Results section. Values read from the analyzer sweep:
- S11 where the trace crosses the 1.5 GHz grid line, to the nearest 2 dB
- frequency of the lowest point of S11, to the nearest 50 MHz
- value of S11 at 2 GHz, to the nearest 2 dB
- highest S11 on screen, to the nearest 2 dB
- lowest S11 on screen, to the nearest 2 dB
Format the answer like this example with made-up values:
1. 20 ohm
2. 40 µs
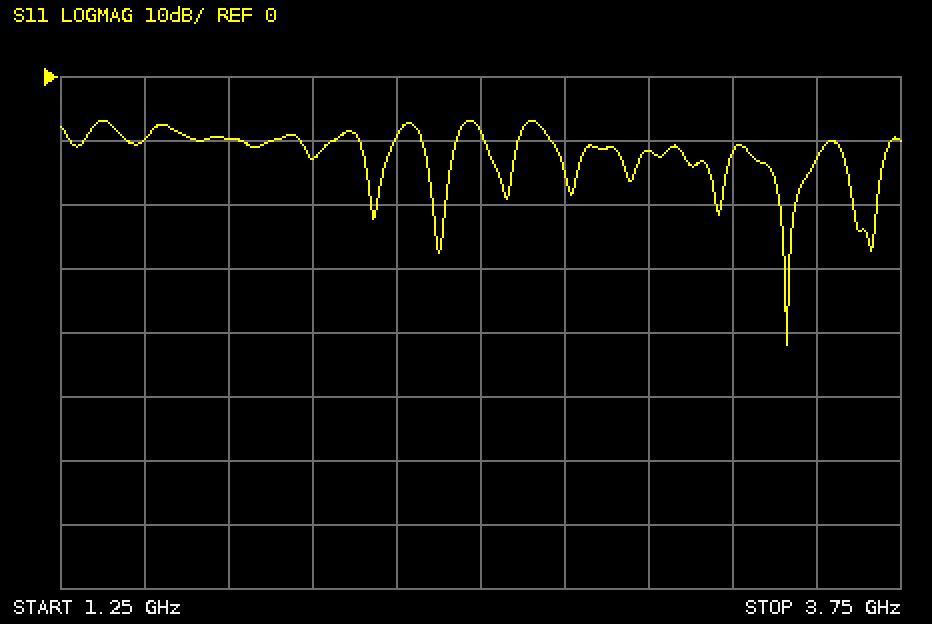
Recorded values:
1. -10 dB
2. 3.40 GHz
3. -12 dB
4. -6 dB
5. -42 dB
